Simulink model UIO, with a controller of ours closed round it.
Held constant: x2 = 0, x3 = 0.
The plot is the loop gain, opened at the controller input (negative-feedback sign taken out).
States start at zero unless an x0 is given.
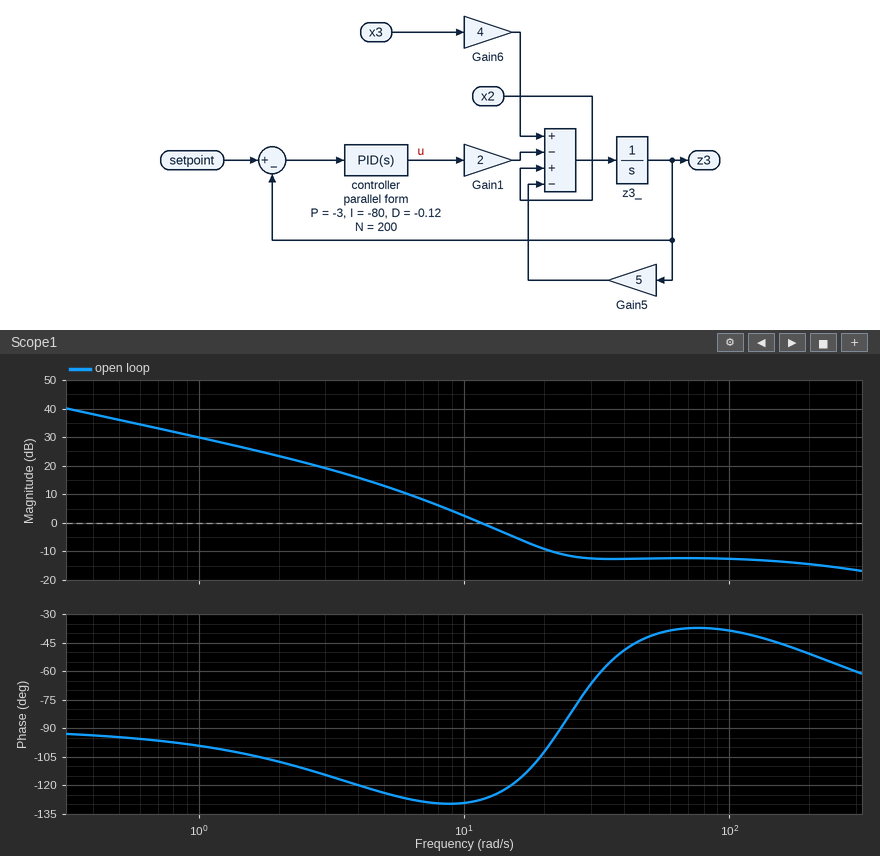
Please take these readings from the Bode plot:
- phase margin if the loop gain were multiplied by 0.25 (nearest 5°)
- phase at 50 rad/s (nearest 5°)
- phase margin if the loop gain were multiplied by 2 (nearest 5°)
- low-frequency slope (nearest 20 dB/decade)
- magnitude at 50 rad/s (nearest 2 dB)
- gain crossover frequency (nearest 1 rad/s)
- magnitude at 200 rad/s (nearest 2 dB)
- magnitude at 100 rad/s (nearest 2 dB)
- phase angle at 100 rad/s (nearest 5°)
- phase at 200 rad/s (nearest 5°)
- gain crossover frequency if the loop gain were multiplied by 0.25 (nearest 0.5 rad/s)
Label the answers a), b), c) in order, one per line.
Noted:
a) 55°
b) -40°
c) 65°
d) -20 dB/decade
e) -12 dB
f) 12 rad/s
g) -14 dB
h) -12 dB
i) -40°
j) -50°
k) 5.5 rad/s
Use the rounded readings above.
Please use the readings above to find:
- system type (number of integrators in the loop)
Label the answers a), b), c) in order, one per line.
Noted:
a) 1
